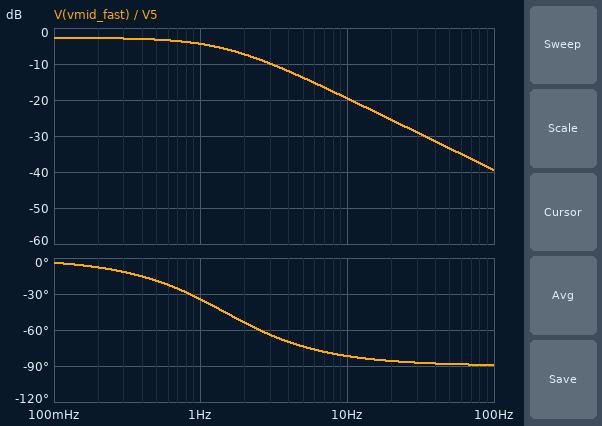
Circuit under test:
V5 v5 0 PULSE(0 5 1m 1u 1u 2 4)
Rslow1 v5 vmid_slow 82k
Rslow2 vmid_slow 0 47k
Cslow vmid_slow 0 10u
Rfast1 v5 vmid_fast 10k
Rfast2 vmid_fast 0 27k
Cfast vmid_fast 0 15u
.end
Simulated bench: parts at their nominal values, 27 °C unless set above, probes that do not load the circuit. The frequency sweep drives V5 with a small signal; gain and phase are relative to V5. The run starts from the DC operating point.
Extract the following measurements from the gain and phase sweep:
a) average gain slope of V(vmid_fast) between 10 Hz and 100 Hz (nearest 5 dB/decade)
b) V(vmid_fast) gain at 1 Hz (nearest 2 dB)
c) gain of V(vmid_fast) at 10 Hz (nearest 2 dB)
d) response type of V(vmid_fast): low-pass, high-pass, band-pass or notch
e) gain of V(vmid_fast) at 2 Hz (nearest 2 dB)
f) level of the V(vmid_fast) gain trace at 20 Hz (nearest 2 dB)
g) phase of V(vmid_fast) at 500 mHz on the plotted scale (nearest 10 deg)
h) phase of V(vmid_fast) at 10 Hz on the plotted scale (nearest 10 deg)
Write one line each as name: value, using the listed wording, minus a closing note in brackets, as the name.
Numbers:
average gain slope of V(vmid_fast) between 10 Hz and 100 Hz: -20 dB/decade
V(vmid_fast) gain at 1 Hz: -4 dB
gain of V(vmid_fast) at 10 Hz: -20 dB
response type of V(vmid_fast): low-pass, high-pass, band-pass or notch: low-pass
gain of V(vmid_fast) at 2 Hz: -8 dB
level of the V(vmid_fast) gain trace at 20 Hz: -26 dB
phase of V(vmid_fast) at 500 mHz on the plotted scale: -20 deg
phase of V(vmid_fast) at 10 Hz on the plotted scale: -80 deg
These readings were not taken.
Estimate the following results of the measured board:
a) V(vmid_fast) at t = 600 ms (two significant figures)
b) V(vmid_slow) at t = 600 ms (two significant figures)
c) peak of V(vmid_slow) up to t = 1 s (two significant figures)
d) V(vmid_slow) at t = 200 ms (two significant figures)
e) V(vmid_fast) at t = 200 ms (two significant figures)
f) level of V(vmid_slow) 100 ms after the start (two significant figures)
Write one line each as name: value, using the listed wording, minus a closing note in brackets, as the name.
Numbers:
V(vmid_fast) at t = 600 ms: 3.6 V
V(vmid_slow) at t = 600 ms: 1.6 V
peak of V(vmid_slow) up to t = 1 s: 1.8 V
V(vmid_slow) at t = 200 ms: 890 mV
V(vmid_fast) at t = 200 ms: 3.1 V
level of V(vmid_slow) 100 ms after the start: 510 mV
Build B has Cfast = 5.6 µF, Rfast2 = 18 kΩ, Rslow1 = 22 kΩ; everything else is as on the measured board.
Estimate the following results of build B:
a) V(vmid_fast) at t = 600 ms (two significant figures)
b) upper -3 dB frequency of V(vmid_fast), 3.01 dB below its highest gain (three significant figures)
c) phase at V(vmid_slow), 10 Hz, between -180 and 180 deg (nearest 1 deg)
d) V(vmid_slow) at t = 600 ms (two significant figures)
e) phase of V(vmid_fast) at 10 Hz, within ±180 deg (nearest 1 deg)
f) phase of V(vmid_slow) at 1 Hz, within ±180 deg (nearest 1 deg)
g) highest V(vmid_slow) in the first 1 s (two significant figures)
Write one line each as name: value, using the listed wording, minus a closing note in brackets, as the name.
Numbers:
V(vmid_fast) at t = 600 ms: 3.2 V
upper -3 dB frequency of V(vmid_fast), 3.01 dB below its highest gain: 4.42 Hz
phase at V(vmid_slow), 10 Hz, between -180 and 180 deg: -84 deg
V(vmid_slow) at t = 600 ms: 3.3 V
phase of V(vmid_fast) at 10 Hz, within ±180 deg: -66 deg
phase of V(vmid_slow) at 1 Hz, within ±180 deg: -43 deg
highest V(vmid_slow) in the first 1 s: 3.4 V
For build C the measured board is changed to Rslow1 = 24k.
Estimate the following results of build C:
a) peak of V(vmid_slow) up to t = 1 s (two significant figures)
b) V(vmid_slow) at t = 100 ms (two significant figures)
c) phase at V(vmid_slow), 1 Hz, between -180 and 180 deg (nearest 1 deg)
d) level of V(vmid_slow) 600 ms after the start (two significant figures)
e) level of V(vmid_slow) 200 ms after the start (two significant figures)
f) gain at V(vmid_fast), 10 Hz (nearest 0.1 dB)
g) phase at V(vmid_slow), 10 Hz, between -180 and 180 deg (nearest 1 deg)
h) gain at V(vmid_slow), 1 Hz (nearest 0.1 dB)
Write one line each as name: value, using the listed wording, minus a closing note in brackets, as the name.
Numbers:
peak of V(vmid_slow) up to t = 1 s: 3.3 V
V(vmid_slow) at t = 100 ms: 1.5 V
phase at V(vmid_slow), 1 Hz, between -180 and 180 deg: -45 deg
level of V(vmid_slow) 600 ms after the start: 3.2 V
level of V(vmid_slow) 200 ms after the start: 2.4 V
gain at V(vmid_fast), 10 Hz: -19.6 dB
phase at V(vmid_slow), 10 Hz, between -180 and 180 deg: -84 deg
gain at V(vmid_slow), 1 Hz: -6.6 dB
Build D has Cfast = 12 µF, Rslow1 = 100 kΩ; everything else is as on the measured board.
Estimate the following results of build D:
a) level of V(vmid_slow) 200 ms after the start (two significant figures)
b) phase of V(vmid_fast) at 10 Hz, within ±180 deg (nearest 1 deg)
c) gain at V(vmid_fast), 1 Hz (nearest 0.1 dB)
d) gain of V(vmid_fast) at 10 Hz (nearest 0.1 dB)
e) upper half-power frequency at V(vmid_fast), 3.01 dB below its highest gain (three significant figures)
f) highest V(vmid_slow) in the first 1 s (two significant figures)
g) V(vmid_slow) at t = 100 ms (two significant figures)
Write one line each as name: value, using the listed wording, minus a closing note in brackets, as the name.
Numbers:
level of V(vmid_slow) 200 ms after the start: 740 mV
phase of V(vmid_fast) at 10 Hz, within ±180 deg: -80 deg
gain at V(vmid_fast), 1 Hz: -3.9 dB
gain of V(vmid_fast) at 10 Hz: -17.7 dB
upper half-power frequency at V(vmid_fast), 3.01 dB below its highest gain: 1.82 Hz
highest V(vmid_slow) in the first 1 s: 1.5 V
V(vmid_slow) at t = 100 ms: 430 mV
